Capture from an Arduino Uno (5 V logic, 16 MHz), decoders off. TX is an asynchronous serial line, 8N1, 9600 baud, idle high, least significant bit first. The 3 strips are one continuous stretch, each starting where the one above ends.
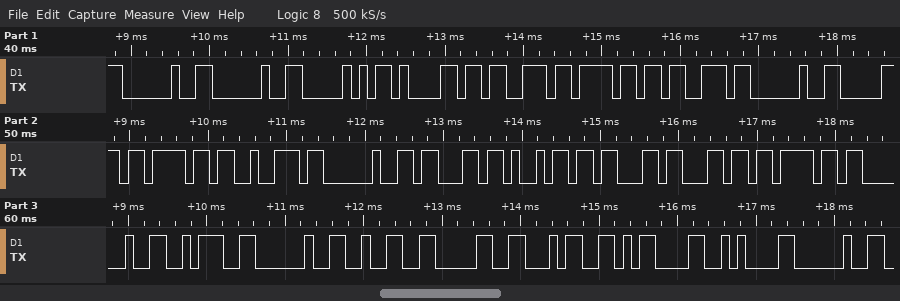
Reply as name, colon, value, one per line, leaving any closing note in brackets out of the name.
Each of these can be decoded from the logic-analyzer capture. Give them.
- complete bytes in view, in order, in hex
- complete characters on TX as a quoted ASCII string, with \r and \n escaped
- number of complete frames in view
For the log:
complete bytes in view, in order, in hex: 20 20 50 61 73 6F 73 20 70 6F 72 20 63 69 63 6C 6F 20 3A 20 32 30 34 0D 0A 20
complete characters on TX as a quoted ASCII string, with \r and \n escaped: "  Pasos por ciclo : 204\r\n "
number of complete frames in view: 26
